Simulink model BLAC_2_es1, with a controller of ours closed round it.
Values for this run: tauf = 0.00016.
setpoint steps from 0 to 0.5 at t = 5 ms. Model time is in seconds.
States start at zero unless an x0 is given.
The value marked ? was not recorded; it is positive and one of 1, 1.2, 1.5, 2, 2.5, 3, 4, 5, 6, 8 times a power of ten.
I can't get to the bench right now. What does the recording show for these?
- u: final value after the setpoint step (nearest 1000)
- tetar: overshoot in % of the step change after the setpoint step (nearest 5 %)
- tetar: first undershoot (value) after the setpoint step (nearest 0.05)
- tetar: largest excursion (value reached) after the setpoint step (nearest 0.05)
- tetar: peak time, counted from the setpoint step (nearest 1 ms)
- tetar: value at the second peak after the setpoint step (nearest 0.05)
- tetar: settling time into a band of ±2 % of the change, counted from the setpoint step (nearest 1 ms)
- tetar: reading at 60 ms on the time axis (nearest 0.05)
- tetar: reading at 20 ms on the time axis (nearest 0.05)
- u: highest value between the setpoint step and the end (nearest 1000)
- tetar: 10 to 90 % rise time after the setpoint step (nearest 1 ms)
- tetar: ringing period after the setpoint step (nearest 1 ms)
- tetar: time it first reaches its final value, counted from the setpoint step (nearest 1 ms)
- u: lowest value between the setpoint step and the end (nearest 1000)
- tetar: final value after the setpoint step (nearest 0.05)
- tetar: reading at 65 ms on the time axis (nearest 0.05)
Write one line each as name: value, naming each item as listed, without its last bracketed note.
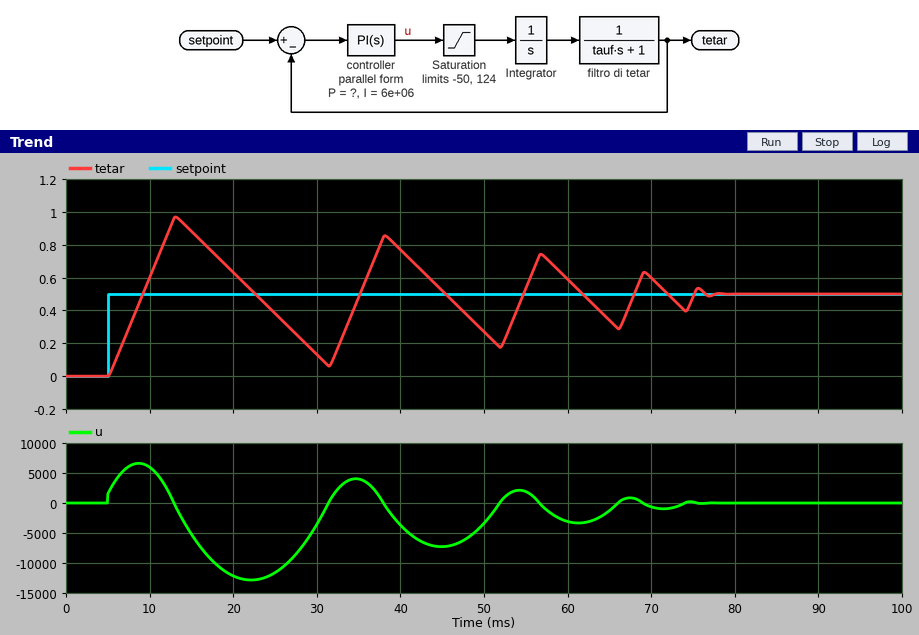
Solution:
u: final value after the setpoint step: 0
tetar: overshoot in % of the step change after the setpoint step: 95 %
tetar: first undershoot (value) after the setpoint step: 0.05
tetar: largest excursion (value reached) after the setpoint step: 0.95
tetar: peak time, counted from the setpoint step: 8 ms
tetar: value at the second peak after the setpoint step: 0.85
tetar: settling time into a band of ±2 % of the change, counted from the setpoint step: 72 ms
tetar: reading at 60 ms on the time axis: 0.60
tetar: reading at 20 ms on the time axis: 0.65
u: highest value between the setpoint step and the end: 7000
tetar: 10 to 90 % rise time after the setpoint step: 3 ms
tetar: ringing period after the setpoint step: 25 ms
tetar: time it first reaches its final value, counted from the setpoint step: 4 ms
u: lowest value between the setpoint step and the end: -13000
tetar: final value after the setpoint step: 0.50
tetar: reading at 65 ms on the time axis: 0.35
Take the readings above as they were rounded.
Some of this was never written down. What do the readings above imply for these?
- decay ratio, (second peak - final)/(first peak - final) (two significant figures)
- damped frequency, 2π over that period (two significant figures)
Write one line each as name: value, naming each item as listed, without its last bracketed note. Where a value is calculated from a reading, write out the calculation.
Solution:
decay ratio, (second peak - final)/(first peak - final): (0.85 - 0.5) / (0.95 - 0.5) = 0.78
damped frequency, 2π over that period: 2π / 25 = 0.25 rad/ms
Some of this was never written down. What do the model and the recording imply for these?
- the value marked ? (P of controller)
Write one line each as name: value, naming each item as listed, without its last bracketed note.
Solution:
the value marked ?: 3000
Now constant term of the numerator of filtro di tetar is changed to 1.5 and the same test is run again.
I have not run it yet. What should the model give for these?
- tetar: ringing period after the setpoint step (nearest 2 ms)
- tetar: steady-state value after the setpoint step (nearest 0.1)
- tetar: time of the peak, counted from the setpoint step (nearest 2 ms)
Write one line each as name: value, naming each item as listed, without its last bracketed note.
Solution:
tetar: ringing period after the setpoint step: 16 ms
tetar: steady-state value after the setpoint step: 0.5
tetar: time of the peak, counted from the setpoint step: 6 ms
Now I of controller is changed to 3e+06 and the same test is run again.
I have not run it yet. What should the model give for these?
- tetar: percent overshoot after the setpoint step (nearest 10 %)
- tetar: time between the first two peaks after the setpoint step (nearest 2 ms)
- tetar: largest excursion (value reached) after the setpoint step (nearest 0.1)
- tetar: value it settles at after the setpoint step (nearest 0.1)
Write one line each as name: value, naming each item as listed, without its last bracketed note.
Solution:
tetar: percent overshoot after the setpoint step: 80 %
tetar: time between the first two peaks after the setpoint step: 20 ms
tetar: largest excursion (value reached) after the setpoint step: 0.9
tetar: value it settles at after the setpoint step: 0.5
